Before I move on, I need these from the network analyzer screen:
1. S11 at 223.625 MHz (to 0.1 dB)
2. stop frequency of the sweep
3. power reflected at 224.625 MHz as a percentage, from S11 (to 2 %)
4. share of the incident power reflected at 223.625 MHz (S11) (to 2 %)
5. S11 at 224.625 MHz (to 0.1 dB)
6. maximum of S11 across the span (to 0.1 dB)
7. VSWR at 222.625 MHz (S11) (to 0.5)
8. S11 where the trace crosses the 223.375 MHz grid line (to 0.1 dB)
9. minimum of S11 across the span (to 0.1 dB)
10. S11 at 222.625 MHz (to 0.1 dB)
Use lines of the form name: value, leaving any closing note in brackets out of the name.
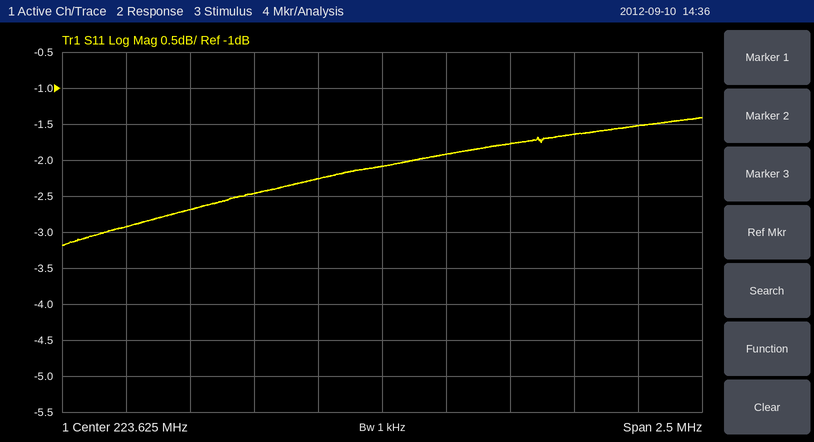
S11 at 223.625 MHz: -2.1 dB
stop frequency of the sweep: 224.875 MHz
power reflected at 224.625 MHz as a percentage, from S11: 70 %
share of the incident power reflected at 223.625 MHz (S11): 62 %
S11 at 224.625 MHz: -1.5 dB
maximum of S11 across the span: -1.4 dB
VSWR at 222.625 MHz (S11): 6.0
S11 where the trace crosses the 223.375 MHz grid line: -2.3 dB
minimum of S11 across the span: -3.2 dB
S11 at 222.625 MHz: -2.9 dB
